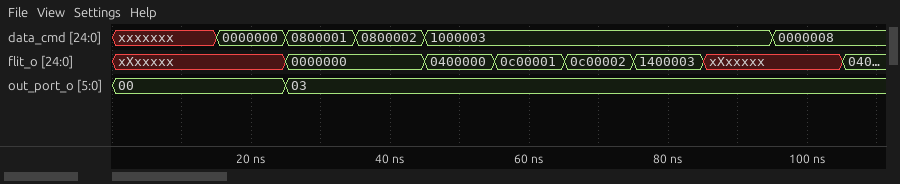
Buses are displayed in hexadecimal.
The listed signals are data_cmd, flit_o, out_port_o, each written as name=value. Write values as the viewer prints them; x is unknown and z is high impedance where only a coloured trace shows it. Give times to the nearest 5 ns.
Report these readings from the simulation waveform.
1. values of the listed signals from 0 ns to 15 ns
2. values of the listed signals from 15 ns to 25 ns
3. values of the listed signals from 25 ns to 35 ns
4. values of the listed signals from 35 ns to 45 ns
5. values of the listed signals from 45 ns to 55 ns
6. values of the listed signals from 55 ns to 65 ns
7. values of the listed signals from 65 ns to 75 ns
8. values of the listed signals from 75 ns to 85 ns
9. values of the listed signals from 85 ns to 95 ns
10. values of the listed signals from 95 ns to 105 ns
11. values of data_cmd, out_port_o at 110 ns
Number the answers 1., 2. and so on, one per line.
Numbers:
1. data_cmd=xxxxxxx, flit_o=xXxxxxx, out_port_o=00
2. data_cmd=0000000, flit_o=xXxxxxx, out_port_o=00
3. data_cmd=0800001, flit_o=0000000, out_port_o=03
4. data_cmd=0800002, flit_o=0000000, out_port_o=03
5. data_cmd=1000003, flit_o=0400000, out_port_o=03
6. data_cmd=1000003, flit_o=0c00001, out_port_o=03
7. data_cmd=1000003, flit_o=0c00002, out_port_o=03
8. data_cmd=1000003, flit_o=1400003, out_port_o=03
9. data_cmd=1000003, flit_o=xXxxxxx, out_port_o=03
10. data_cmd=0000008, flit_o=xXxxxxx, out_port_o=03
11. data_cmd=0000008, out_port_o=03
